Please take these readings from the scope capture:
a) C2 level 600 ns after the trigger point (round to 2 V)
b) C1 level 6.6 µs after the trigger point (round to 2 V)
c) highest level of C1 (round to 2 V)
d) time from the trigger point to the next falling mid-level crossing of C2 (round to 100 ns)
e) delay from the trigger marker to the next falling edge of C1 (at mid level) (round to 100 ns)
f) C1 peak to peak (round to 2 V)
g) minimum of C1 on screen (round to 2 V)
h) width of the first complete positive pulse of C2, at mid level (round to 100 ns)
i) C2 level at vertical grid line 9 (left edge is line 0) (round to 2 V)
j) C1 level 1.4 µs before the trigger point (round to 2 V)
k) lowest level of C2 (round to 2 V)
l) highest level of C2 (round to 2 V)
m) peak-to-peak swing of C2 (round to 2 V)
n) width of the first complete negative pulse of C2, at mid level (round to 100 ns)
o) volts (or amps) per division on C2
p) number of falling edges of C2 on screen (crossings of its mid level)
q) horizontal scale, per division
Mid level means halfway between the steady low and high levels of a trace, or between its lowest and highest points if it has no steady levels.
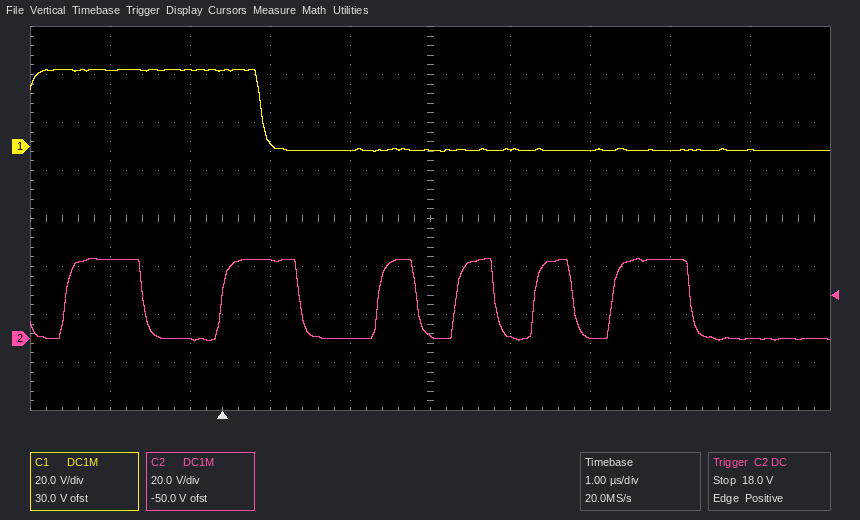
32 V
-2 V
32 V
1.0 µs
500 ns
34 V
-2 V
1.0 µs
0 V
32 V
0 V
34 V
34 V
1.0 µs
20 V
6
1 µs
